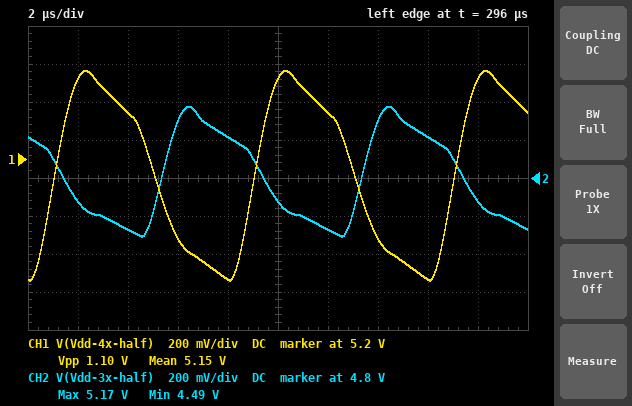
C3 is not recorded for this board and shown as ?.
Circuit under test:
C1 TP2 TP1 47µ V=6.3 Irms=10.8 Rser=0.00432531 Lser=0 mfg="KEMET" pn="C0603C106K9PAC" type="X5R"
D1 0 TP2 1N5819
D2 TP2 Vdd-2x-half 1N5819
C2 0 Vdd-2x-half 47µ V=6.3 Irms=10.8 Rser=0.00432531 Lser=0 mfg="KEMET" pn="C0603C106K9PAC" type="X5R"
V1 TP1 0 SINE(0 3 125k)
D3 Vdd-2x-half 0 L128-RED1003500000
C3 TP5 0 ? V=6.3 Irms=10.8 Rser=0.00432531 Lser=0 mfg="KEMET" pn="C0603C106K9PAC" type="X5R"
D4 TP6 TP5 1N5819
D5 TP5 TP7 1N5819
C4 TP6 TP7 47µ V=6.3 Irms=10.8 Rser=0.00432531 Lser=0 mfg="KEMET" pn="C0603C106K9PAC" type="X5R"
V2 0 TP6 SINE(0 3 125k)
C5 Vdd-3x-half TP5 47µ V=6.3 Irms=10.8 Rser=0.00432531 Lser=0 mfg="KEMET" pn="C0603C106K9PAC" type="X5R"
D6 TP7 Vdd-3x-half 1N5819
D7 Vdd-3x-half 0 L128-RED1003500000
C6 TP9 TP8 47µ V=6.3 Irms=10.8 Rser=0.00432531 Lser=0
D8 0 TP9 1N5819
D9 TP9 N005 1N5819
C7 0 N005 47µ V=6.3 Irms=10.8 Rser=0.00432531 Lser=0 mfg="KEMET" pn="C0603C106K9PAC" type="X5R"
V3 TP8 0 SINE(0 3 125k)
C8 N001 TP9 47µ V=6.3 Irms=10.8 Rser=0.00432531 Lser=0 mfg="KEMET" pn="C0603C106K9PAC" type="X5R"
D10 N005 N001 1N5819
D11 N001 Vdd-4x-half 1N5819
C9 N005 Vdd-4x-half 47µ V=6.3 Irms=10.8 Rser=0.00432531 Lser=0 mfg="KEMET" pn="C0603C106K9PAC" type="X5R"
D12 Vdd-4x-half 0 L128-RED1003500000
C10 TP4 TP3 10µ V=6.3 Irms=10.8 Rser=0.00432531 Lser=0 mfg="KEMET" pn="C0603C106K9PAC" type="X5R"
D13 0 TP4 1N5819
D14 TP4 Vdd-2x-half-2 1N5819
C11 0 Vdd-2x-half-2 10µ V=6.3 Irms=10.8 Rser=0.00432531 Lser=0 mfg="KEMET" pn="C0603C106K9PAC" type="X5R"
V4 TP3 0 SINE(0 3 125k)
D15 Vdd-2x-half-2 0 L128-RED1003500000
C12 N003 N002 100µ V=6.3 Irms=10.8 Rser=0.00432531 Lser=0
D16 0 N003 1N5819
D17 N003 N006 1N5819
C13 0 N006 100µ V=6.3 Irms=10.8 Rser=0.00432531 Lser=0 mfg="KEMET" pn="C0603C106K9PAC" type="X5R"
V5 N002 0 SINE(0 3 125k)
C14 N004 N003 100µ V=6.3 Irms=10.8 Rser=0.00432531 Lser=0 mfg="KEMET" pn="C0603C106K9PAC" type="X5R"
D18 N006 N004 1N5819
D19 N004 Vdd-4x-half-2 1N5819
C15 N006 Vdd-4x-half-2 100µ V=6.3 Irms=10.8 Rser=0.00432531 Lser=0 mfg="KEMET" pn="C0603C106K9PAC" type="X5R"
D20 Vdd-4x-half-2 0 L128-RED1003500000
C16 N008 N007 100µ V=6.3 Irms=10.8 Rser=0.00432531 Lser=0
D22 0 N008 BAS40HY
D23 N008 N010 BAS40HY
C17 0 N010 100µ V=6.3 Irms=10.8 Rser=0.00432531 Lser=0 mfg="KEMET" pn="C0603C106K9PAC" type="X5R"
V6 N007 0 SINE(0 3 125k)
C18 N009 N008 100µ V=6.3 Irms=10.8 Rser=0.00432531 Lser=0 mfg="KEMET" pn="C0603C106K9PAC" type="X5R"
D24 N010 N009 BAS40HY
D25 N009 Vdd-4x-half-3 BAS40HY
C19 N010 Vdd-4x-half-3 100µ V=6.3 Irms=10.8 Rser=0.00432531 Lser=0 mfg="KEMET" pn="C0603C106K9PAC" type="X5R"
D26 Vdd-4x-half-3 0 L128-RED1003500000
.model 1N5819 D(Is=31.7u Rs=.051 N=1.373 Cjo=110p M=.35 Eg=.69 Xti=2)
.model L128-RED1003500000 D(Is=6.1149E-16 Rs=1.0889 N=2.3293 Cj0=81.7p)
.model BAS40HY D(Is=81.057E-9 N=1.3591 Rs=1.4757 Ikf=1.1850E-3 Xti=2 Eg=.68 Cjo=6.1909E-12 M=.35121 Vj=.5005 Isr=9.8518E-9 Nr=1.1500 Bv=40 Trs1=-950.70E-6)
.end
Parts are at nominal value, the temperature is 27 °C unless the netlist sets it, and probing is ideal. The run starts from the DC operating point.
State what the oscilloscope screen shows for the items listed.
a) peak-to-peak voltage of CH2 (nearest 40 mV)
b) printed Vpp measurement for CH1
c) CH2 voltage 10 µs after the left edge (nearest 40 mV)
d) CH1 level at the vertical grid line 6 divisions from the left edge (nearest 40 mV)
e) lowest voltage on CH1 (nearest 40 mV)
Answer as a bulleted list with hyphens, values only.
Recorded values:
- 680 mV
- 1.10 V
- 4.68 V
- 5.44 V
- 4.56 V
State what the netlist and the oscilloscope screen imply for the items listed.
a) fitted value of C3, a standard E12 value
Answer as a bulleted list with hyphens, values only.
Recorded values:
- 100 µF
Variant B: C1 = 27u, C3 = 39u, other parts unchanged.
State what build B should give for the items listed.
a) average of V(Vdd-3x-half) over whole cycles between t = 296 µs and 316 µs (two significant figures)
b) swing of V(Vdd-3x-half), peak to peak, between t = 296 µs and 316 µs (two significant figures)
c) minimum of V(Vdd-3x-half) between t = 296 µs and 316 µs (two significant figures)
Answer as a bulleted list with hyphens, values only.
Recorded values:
- 4.7 V
- 1.1 V
- 4.1 V
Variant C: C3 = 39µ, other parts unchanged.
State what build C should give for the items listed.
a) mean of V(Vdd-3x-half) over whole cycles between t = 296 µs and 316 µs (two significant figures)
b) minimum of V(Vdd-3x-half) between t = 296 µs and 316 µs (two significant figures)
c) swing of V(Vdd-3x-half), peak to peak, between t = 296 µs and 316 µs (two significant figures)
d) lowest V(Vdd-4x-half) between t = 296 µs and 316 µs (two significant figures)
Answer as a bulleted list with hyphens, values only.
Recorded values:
- 4.7 V
- 4.1 V
- 1.1 V
- 4.6 V
